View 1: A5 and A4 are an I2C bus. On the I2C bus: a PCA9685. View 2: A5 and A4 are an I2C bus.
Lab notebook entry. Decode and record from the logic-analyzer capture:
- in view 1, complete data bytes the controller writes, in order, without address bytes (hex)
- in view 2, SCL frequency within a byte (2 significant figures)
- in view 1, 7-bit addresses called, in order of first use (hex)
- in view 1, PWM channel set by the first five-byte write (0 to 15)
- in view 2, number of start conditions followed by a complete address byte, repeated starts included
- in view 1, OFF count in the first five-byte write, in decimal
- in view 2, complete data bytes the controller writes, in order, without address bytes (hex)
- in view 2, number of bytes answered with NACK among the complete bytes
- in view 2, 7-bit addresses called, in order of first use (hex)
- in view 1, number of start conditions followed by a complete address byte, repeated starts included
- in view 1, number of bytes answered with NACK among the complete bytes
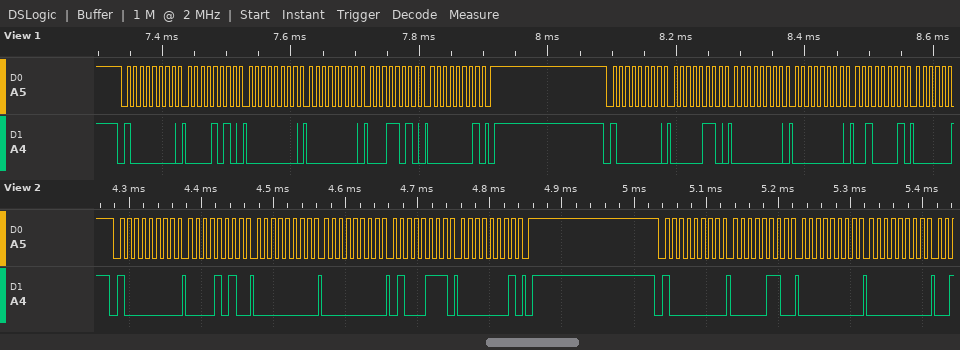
0A 00 00 1A 01 06 00 00 21
100 kHz
0x40
1
2
282
0A 00 00 47 01 06 00 00
0
0x40
2
0
